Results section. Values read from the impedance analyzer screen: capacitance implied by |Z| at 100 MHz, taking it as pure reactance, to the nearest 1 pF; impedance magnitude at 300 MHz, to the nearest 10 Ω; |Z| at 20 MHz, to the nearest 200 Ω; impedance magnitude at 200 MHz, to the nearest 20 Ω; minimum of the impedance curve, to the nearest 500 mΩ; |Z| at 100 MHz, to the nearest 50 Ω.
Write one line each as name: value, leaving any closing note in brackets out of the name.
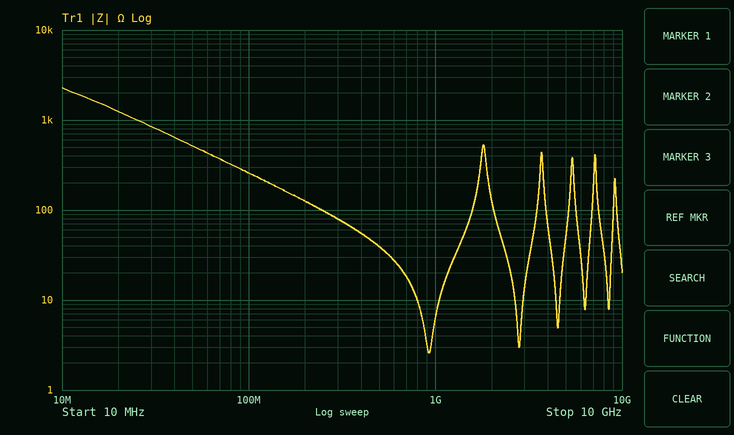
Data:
capacitance implied by |Z| at 100 MHz, taking it as pure reactance, to the nearest 1 pF: 6 pF
impedance magnitude at 300 MHz, to the nearest 10 Ω: 80 Ω
|Z| at 20 MHz, to the nearest 200 Ω: 1.2 kΩ
impedance magnitude at 200 MHz, to the nearest 20 Ω: 120 Ω
minimum of the impedance curve, to the nearest 500 mΩ: 2.5 Ω
|Z| at 100 MHz, to the nearest 50 Ω: 250 Ω
